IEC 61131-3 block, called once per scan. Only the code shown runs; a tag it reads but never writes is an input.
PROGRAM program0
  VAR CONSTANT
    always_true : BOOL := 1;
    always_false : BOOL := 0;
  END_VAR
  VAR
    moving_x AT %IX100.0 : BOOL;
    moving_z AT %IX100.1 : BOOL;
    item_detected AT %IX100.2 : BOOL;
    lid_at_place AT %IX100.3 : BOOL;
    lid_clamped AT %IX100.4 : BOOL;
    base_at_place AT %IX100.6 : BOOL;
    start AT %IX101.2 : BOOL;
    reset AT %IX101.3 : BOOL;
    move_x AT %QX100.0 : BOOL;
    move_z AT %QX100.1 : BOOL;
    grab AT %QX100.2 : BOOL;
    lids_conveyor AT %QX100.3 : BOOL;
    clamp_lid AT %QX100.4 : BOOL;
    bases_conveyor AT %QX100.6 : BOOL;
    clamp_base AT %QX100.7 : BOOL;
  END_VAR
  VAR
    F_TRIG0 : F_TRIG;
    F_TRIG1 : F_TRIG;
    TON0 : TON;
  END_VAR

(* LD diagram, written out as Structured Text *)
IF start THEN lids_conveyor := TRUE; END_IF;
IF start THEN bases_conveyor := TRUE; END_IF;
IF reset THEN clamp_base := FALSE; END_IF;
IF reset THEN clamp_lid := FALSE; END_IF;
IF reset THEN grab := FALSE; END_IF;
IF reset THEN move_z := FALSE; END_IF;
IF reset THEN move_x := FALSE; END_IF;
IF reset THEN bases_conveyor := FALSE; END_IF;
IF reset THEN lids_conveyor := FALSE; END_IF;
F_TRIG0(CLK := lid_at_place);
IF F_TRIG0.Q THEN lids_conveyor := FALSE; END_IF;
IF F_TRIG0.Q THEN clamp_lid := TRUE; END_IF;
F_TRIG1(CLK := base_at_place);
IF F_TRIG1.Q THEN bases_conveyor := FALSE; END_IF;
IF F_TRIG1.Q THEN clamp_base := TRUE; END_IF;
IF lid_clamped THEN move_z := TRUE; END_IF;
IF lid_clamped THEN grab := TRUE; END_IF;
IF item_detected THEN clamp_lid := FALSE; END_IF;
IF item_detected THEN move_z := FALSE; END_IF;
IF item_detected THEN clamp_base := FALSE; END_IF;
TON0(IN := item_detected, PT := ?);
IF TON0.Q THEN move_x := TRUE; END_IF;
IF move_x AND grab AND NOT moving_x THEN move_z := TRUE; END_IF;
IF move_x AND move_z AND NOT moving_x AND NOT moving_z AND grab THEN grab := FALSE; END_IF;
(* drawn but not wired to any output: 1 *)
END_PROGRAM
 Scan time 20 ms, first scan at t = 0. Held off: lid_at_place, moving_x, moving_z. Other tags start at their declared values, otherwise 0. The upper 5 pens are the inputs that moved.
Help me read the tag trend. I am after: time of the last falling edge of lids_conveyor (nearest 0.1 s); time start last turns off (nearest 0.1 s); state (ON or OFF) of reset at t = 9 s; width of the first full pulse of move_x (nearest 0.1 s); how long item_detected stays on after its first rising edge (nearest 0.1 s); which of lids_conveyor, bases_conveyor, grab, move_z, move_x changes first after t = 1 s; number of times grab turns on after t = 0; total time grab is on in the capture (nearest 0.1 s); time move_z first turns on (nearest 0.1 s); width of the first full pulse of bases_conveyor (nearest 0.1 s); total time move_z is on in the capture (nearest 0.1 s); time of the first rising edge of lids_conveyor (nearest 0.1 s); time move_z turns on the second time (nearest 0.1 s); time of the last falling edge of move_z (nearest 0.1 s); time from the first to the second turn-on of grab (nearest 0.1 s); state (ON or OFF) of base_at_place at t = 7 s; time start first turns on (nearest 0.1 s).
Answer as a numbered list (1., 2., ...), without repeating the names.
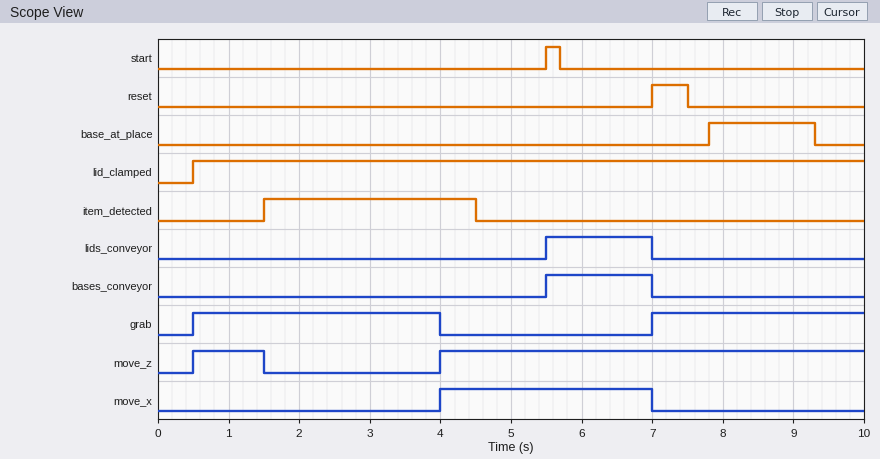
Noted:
1. 7.0 s
2. 5.7 s
3. OFF
4. 3.0 s
5. 3.0 s
6. move_z
7. 2
8. 6.5 s
9. 0.5 s
10. 1.5 s
11. 7.0 s
12. 5.5 s
13. 4.0 s
14. 1.5 s
15. 6.5 s
16. OFF
17. 5.5 s
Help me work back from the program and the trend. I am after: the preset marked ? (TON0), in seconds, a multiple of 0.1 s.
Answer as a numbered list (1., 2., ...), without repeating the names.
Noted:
1. 2.5 s
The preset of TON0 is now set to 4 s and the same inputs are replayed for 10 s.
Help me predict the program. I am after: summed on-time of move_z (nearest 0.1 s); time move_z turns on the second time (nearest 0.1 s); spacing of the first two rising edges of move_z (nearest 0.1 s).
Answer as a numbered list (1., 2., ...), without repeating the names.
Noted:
1. 6.5 s
2. 4.5 s
3. 4.0 s
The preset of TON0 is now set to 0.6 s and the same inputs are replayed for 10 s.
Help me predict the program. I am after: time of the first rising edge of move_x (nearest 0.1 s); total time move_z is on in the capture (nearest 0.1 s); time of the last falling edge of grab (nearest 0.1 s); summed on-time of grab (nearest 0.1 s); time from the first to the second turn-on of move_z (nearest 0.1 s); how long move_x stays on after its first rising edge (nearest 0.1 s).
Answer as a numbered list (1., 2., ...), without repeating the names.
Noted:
1. 2.1 s
2. 8.9 s
3. 2.1 s
4. 4.6 s
5. 1.6 s
6. 4.9 s
